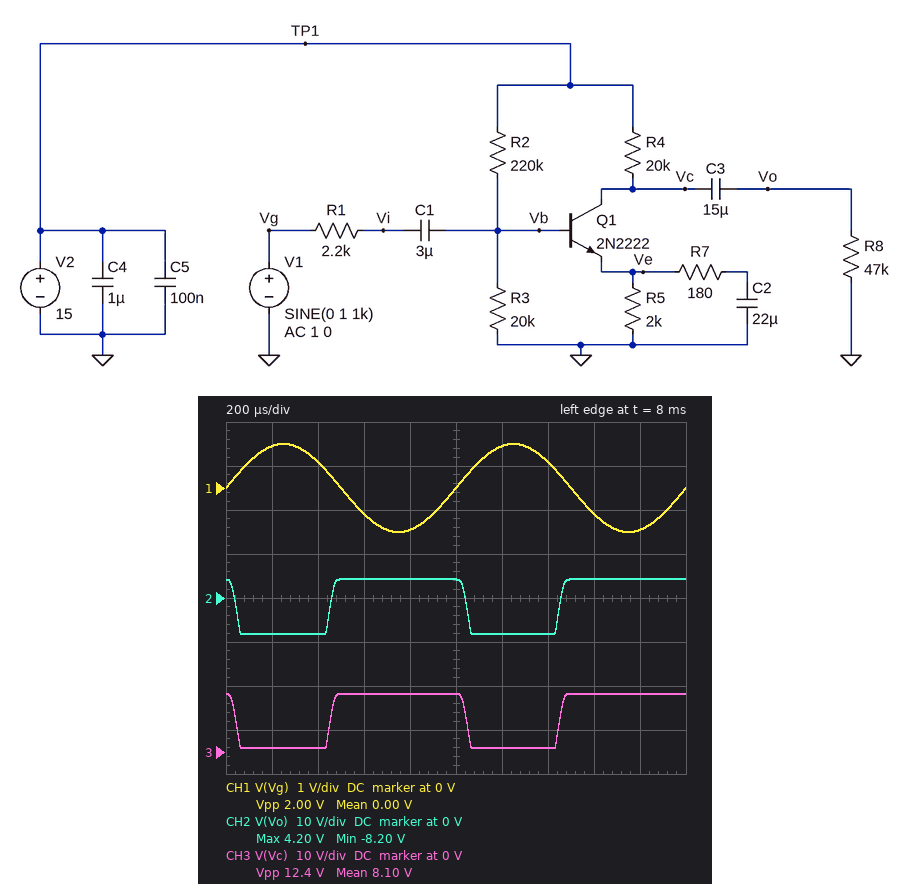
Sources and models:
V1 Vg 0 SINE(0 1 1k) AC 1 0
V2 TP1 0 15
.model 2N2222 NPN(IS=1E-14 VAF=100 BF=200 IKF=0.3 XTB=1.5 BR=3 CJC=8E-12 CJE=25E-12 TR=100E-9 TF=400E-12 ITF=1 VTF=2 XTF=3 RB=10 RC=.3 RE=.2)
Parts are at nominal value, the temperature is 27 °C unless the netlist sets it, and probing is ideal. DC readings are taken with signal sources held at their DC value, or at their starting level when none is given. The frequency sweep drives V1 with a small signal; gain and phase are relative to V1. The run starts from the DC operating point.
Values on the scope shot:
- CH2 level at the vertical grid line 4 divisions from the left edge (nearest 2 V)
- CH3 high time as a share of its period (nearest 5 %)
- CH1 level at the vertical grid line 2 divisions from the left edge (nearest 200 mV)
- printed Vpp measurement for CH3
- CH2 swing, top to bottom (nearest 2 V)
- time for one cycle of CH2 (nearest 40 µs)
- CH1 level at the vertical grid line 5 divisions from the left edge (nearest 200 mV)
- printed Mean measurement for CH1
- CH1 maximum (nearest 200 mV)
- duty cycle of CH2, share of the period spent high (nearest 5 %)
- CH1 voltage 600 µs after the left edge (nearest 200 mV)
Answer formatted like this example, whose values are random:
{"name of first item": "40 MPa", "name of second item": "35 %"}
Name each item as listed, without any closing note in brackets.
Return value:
{"CH2 level at the vertical grid line 4 divisions from the left edge": "4 V", "CH3 high time as a share of its period": "60 %", "CH1 level at the vertical grid line 2 divisions from the left edge": "600 mV", "printed Vpp measurement for CH3": "12.4 V", "CH2 swing, top to bottom": "12 V", "time for one cycle of CH2": "1.00 ms", "CH1 level at the vertical grid line 5 divisions from the left edge": "0 V", "printed Mean measurement for CH1": "0.00 V", "CH1 maximum": "1.0 V", "duty cycle of CH2, share of the period spent high": "60 %", "CH1 voltage 600 µs after the left edge": "-600 mV"}
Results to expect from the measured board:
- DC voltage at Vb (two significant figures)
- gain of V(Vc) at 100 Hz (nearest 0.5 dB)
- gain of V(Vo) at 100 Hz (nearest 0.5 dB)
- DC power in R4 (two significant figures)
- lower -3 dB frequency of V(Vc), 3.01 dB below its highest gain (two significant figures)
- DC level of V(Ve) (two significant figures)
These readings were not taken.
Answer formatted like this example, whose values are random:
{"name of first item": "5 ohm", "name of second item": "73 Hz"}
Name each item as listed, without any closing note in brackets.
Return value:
{"DC voltage at Vb": "1.2 V", "gain of V(Vc) at 100 Hz": "33.0 dB", "gain of V(Vo) at 100 Hz": "33.0 dB", "DC power in R4": "1.8 mW", "lower -3 dB frequency of V(Vc), 3.01 dB below its highest gain": "27 Hz", "DC level of V(Ve)": "600 mV"}
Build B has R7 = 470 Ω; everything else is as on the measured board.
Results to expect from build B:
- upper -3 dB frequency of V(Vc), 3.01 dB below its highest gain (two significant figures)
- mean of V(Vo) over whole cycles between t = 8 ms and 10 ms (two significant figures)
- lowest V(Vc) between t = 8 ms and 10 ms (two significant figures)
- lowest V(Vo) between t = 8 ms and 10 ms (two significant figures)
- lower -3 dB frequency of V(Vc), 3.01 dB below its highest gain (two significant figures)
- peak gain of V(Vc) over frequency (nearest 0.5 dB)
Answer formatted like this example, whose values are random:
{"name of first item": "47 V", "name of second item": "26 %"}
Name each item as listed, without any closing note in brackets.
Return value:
{"upper -3 dB frequency of V(Vc), 3.01 dB below its highest gain": "570 kHz", "mean of V(Vo) over whole cycles between t = 8 ms and 10 ms": "-950 mV", "lowest V(Vc) between t = 8 ms and 10 ms": "930 mV", "lowest V(Vo) between t = 8 ms and 10 ms": "-8.1 V", "lower -3 dB frequency of V(Vc), 3.01 dB below its highest gain": "13 Hz", "peak gain of V(Vc) over frequency": "28.5 dB"}
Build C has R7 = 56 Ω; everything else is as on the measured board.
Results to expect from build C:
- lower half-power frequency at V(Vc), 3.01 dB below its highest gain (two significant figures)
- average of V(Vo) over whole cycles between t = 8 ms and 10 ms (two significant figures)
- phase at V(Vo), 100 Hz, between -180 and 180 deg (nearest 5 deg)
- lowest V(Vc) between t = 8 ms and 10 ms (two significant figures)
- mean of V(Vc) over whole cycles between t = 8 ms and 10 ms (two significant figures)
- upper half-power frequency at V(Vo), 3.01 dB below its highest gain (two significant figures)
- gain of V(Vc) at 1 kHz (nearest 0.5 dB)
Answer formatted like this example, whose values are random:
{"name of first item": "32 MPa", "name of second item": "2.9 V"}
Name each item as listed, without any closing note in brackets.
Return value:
{"lower half-power frequency at V(Vc), 3.01 dB below its highest gain": "49 Hz", "average of V(Vo) over whole cycles between t = 8 ms and 10 ms": "-790 mV", "phase at V(Vo), 100 Hz, between -180 and 180 deg": "-155 deg", "lowest V(Vc) between t = 8 ms and 10 ms": "730 mV", "mean of V(Vc) over whole cycles between t = 8 ms and 10 ms": "8.2 V", "upper half-power frequency at V(Vo), 3.01 dB below its highest gain": "210 kHz", "gain of V(Vc) at 1 kHz": "38.0 dB"}
